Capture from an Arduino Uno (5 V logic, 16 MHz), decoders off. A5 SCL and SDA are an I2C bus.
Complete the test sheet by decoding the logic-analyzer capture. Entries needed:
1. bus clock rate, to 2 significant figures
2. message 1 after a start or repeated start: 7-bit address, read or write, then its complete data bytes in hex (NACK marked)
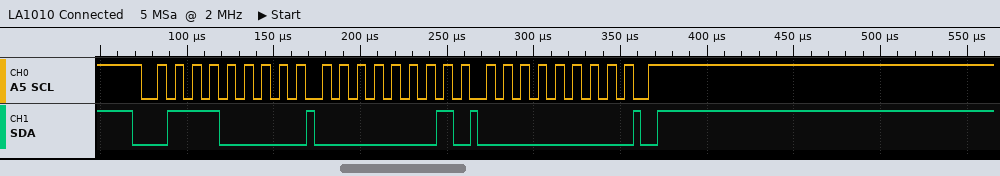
100 kHz
0x38 write: 01 00
